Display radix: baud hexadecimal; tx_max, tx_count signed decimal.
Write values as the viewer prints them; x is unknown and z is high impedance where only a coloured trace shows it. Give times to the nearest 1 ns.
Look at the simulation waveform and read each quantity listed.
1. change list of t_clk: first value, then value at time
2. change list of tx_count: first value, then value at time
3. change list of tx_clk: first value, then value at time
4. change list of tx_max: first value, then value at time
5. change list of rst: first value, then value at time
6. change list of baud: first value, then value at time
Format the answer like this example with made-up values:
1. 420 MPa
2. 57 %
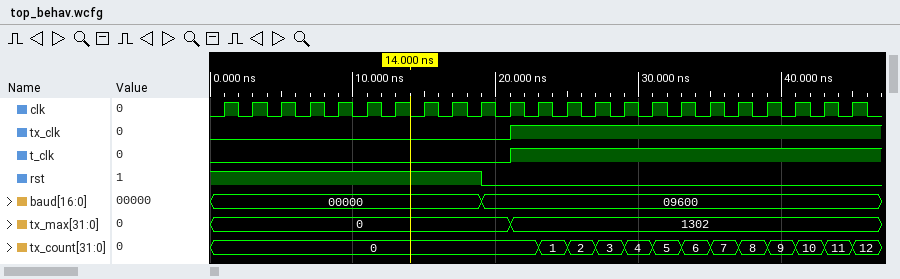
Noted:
1. 0, 1 at 21 ns
2. 0, 1 at 23 ns, 2 at 25 ns, 3 at 27 ns, 4 at 29 ns, 5 at 31 ns, 6 at 33 ns, 7 at 35 ns, 8 at 37 ns, 9 at 39 ns, 10 at 41 ns, 11 at 43 ns, 12 at 45 ns
3. 0, 1 at 21 ns
4. 0, 1302 at 21 ns
5. 1, 0 at 19 ns
6. 00000, 09600 at 19 ns
